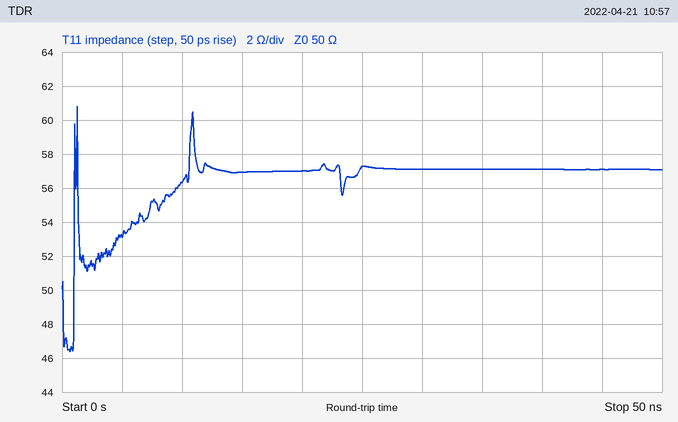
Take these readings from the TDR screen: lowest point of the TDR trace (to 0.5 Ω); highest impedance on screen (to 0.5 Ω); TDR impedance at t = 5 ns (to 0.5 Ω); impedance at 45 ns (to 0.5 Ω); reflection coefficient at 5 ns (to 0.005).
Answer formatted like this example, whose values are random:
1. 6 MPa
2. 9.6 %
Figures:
1. 46.5 Ω
2. 61.0 Ω
3. 53.0 Ω
4. 57.0 Ω
5. +0.030
